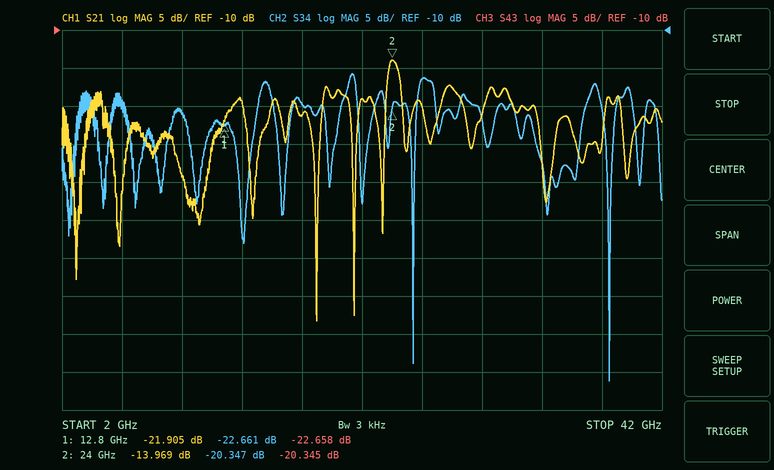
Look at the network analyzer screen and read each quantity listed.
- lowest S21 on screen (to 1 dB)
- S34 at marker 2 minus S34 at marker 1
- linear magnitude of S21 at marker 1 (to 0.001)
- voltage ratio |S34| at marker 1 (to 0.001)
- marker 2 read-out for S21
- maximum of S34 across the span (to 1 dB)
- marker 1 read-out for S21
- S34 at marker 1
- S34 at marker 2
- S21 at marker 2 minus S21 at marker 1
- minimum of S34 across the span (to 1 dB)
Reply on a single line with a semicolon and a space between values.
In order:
-48 dB; 2.314 dB; 0.080; 0.074; -13.969 dB; -16 dB; -21.905 dB; -22.661 dB; -20.347 dB; 7.936 dB; -56 dB
